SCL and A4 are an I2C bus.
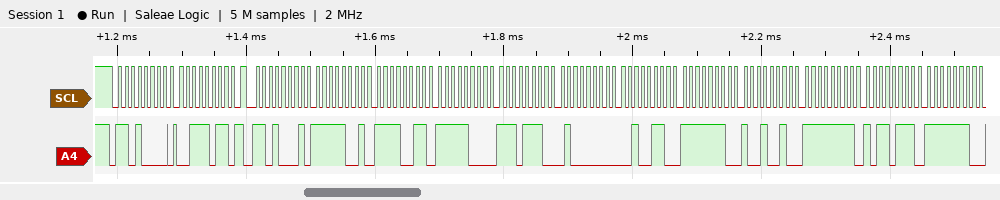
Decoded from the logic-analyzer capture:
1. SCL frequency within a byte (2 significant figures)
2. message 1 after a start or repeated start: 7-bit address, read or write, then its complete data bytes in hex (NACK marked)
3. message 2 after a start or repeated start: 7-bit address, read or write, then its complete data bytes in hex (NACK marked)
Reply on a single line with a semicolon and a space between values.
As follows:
100 kHz; 0x68 write: 3B; 0x68 read: F9 F3 F8 EE 40 26 FE 92 FF B7 FE
